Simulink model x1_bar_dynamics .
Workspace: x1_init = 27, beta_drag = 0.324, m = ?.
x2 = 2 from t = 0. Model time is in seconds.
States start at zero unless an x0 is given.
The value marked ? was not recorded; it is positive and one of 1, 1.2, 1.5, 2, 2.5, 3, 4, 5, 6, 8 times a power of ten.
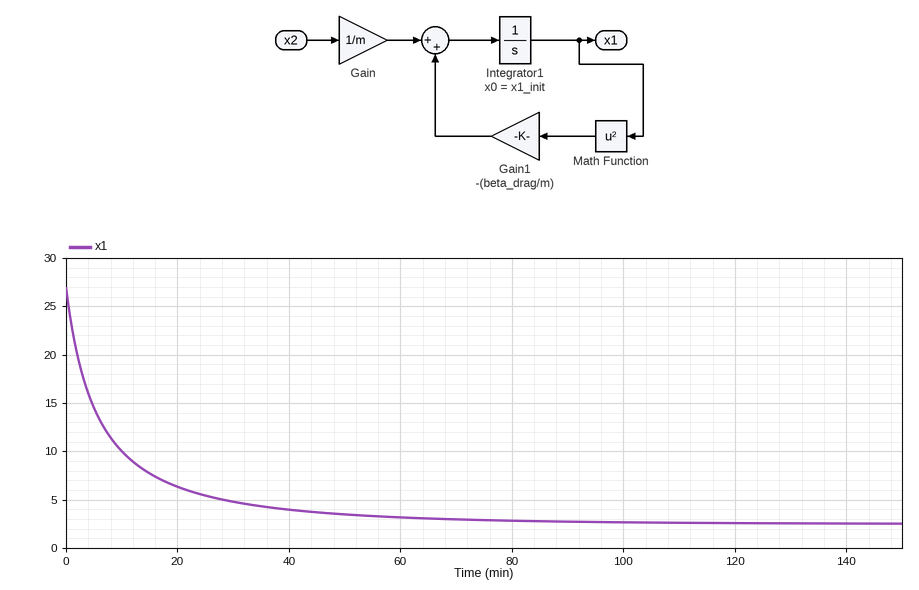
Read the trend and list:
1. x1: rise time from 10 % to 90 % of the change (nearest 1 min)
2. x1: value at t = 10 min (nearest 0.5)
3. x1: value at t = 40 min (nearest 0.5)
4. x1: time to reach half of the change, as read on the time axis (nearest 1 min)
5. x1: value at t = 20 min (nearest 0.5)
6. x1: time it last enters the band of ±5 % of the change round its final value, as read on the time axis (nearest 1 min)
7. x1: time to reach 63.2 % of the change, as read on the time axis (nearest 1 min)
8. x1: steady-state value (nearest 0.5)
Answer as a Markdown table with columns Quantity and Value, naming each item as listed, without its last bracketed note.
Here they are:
| Quantity | Value |
|---|---|
| x1: rise time from 10 % to 90 % of the change | 28 min |
| x1: value at t = 10 min | 10.0 |
| x1: value at t = 40 min | 4.0 |
| x1: time to reach half of the change, as read on the time axis | 5 min |
| x1: value at t = 20 min | 6.5 |
| x1: time it last enters the band of ±5 % of the change round its final value, as read on the time axis | 45 min |
| x1: time to reach 63.2 % of the change, as read on the time axis | 8 min |
| x1: steady-state value | 2.5 |
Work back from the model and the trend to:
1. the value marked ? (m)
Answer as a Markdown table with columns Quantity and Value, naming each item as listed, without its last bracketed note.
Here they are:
| Quantity | Value |
|---|---|
| the value marked ? | 3000 |
